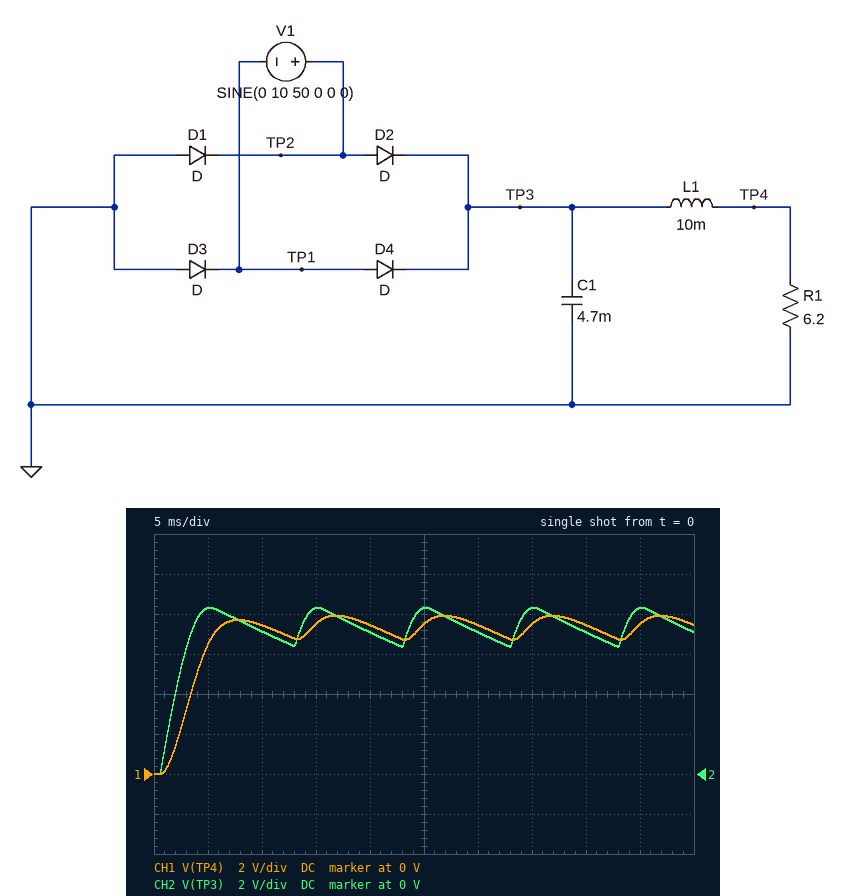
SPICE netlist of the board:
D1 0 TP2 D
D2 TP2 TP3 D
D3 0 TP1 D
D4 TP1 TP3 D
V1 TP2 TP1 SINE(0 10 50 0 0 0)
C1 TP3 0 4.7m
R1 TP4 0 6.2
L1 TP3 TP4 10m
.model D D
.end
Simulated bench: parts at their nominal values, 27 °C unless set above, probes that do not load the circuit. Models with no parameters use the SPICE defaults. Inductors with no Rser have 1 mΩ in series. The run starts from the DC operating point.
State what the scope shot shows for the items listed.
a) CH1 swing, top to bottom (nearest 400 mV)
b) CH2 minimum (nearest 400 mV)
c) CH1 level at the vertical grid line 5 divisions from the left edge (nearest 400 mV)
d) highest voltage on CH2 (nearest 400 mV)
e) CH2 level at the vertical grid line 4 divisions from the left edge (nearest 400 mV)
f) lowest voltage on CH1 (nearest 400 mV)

8.0 V
0 V
7.6 V
8.4 V
7.2 V
0 V
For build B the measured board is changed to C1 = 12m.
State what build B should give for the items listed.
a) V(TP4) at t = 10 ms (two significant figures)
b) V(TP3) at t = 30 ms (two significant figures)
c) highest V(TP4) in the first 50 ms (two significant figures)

7.9 V
7.8 V
8.1 V
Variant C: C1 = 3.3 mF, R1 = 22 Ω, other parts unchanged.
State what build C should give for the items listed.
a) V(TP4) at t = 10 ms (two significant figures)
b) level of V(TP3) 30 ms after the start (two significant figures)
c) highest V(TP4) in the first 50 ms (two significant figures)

7.9 V
7.8 V
8.3 V
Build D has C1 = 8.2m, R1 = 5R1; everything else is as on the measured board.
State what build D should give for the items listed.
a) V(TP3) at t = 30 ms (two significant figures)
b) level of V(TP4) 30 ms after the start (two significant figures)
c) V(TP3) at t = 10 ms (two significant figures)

7.4 V
7.7 V
7.5 V
